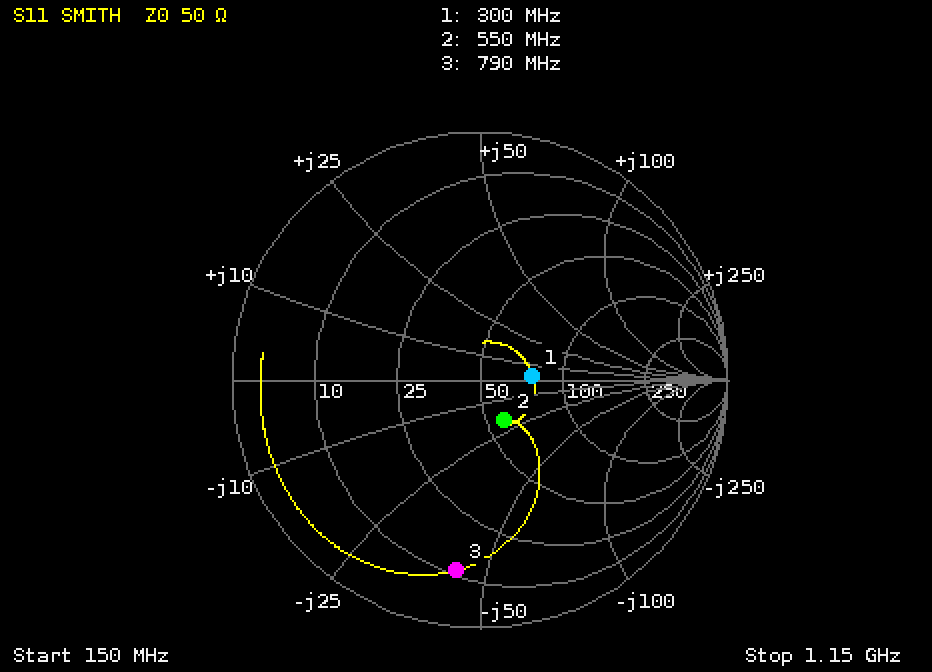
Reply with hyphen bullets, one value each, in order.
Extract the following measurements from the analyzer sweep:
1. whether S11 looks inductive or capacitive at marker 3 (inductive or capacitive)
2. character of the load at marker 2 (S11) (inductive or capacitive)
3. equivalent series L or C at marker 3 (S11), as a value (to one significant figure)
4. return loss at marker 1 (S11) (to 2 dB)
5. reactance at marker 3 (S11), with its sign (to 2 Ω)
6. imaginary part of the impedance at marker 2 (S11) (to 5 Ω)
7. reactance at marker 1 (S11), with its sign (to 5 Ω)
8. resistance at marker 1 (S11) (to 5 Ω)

- capacitive
- capacitive
- 5 pF
- 14 dB
- -42 Ω
- -20 Ω
- +5 Ω
- 75 Ω
